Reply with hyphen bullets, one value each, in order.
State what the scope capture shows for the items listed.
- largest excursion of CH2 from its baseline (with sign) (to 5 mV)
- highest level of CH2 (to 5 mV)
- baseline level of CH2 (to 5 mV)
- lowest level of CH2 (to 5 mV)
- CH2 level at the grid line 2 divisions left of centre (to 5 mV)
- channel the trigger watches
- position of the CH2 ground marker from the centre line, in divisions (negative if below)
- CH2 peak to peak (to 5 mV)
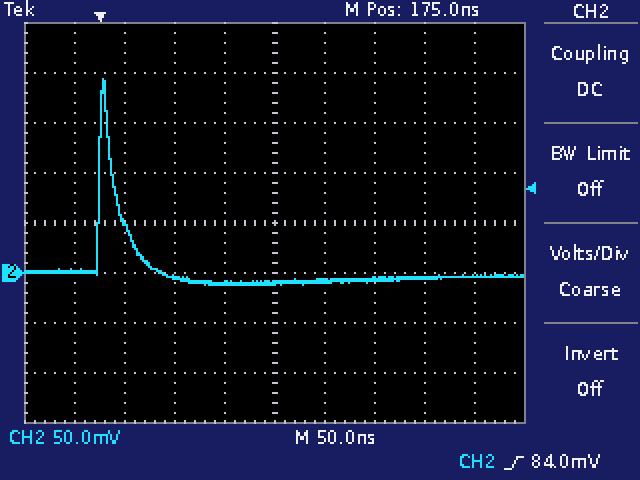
- +200 mV
- 195 mV
- -5 mV
- -10 mV
- -5 mV
- CH2
- -1.0 div
- 205 mV
